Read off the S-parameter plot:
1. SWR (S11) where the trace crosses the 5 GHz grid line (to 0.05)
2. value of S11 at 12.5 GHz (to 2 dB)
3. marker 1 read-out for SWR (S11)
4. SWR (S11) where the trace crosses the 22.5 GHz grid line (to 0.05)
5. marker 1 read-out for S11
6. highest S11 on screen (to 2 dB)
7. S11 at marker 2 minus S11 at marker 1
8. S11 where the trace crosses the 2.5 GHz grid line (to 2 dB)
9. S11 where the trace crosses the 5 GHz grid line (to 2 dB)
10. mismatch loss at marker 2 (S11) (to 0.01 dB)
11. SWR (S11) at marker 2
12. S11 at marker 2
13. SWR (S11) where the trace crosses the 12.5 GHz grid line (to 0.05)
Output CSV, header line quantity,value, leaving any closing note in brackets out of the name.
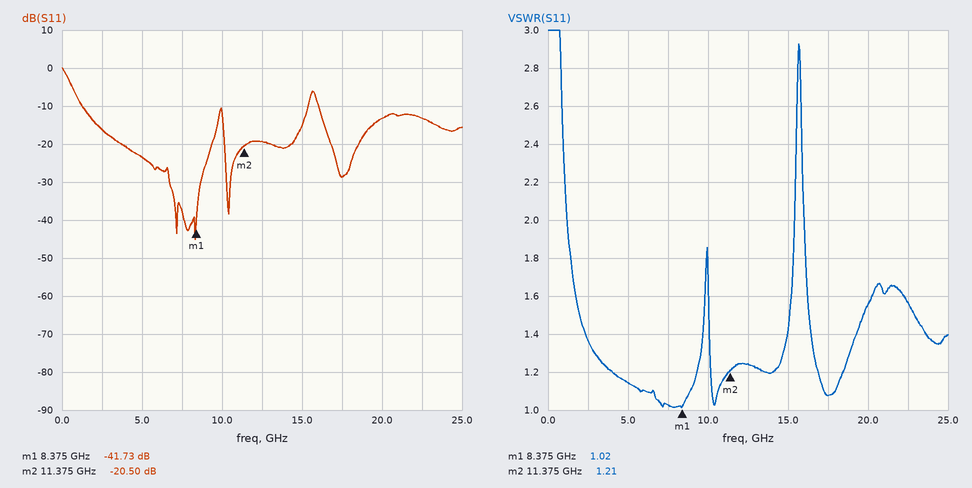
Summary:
quantity,value
SWR (S11) where the trace crosses the 5 GHz grid line,1.15
value of S11 at 12.5 GHz,-20 dB
marker 1 read-out for SWR,1.02
SWR (S11) where the trace crosses the 22.5 GHz grid line,1.55
marker 1 read-out for S11,-41.73 dB
highest S11 on screen,0 dB
S11 at marker 2 minus S11 at marker 1,21.23 dB
S11 where the trace crosses the 2.5 GHz grid line,-16 dB
S11 where the trace crosses the 5 GHz grid line,-24 dB
mismatch loss at marker 2 (S11),0.04 dB
SWR (S11) at marker 2,1.21
S11 at marker 2,-20.50 dB
SWR (S11) where the trace crosses the 12.5 GHz grid line,1.25
